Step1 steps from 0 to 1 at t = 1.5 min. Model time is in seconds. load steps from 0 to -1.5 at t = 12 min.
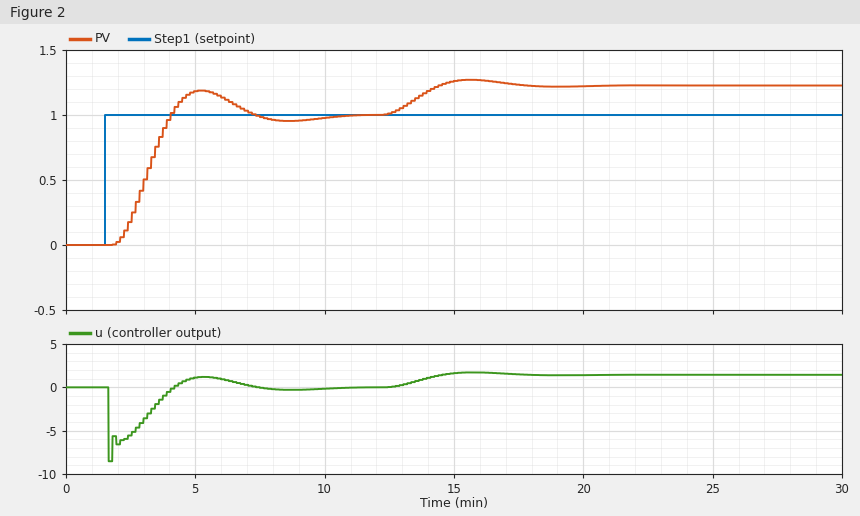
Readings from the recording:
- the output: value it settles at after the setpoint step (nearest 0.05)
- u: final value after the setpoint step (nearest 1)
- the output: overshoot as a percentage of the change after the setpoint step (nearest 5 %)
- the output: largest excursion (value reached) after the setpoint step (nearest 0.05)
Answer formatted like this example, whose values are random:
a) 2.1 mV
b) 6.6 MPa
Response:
a) 1.00
b) 0
c) 20 %
d) 1.20
